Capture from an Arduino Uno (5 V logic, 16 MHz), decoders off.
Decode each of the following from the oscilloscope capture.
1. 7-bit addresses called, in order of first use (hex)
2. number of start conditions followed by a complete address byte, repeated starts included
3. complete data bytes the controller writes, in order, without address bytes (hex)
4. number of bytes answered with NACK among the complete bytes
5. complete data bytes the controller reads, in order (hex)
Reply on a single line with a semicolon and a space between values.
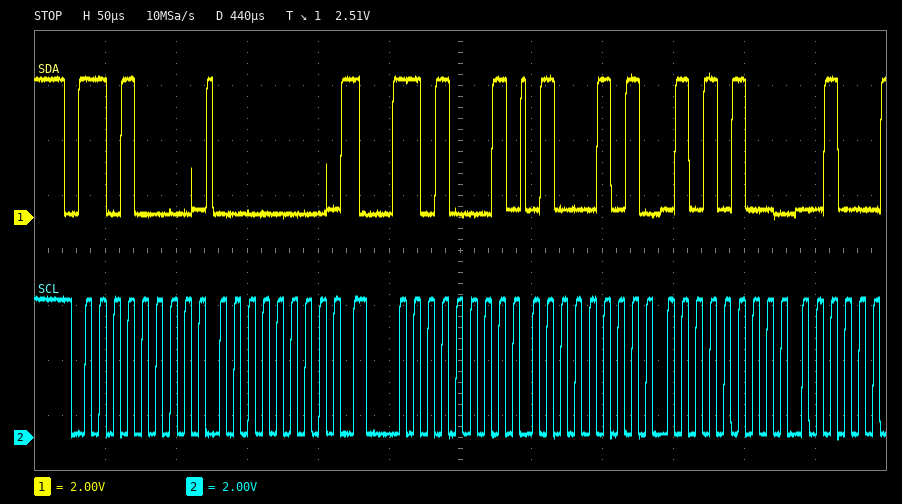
0x68; 2; 00; 0; 45 54
